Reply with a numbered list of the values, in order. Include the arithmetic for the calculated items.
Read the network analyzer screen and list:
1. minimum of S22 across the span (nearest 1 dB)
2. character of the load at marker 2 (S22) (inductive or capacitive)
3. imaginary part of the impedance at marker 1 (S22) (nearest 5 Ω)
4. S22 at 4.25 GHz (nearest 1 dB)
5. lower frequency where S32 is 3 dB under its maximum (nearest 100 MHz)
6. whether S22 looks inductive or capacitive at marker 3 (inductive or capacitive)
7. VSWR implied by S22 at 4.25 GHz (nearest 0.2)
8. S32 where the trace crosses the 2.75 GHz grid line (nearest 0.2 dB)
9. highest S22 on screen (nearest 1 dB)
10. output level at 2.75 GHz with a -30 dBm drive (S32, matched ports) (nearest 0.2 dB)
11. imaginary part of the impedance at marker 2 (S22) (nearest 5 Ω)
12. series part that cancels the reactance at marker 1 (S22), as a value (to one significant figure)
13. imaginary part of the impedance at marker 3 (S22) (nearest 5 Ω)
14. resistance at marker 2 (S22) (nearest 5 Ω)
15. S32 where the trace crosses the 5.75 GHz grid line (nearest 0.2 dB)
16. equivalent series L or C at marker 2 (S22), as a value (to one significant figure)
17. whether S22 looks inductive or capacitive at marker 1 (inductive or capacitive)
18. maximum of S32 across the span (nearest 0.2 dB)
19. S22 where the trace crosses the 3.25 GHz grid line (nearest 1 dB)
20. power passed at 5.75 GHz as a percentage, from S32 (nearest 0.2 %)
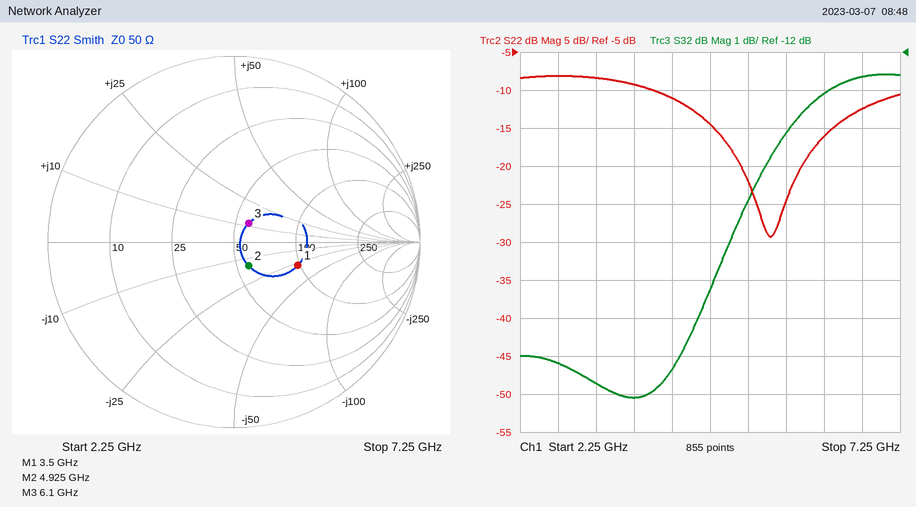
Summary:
1. -29 dB
2. capacitive
3. -30 Ω
4. -11 dB
5. 5.3 GHz
6. inductive
7. |Γ| = 10^(-11/20) = 0.2818; VSWR = (1 + 0.2818)/(1 − 0.2818) ≈ 1.8
8. -20.2 dB
9. -8 dB
10. -30 dBm + (-20.2 dB) = -50.2 dBm
11. -15 Ω
12. L = 30 Ω/(2π × 3.5 GHz) ≈ 1 nH
13. +10 Ω
14. 55 Ω
15. -14.2 dB
16. C = 1/(2π × 4.925 GHz × 15 Ω) ≈ 2 pF
17. capacitive
18. -12.6 dB
19. -8 dB
20. 10^(-14.2/10) ≈ 3.8 %
